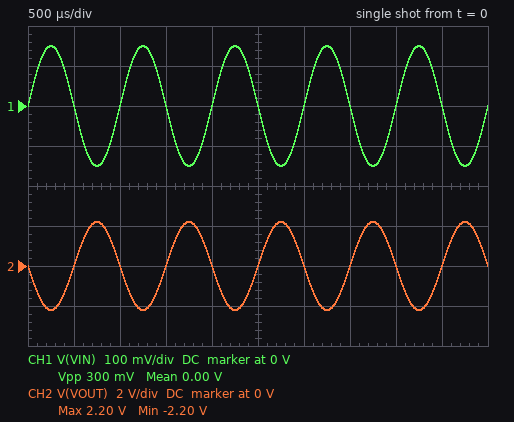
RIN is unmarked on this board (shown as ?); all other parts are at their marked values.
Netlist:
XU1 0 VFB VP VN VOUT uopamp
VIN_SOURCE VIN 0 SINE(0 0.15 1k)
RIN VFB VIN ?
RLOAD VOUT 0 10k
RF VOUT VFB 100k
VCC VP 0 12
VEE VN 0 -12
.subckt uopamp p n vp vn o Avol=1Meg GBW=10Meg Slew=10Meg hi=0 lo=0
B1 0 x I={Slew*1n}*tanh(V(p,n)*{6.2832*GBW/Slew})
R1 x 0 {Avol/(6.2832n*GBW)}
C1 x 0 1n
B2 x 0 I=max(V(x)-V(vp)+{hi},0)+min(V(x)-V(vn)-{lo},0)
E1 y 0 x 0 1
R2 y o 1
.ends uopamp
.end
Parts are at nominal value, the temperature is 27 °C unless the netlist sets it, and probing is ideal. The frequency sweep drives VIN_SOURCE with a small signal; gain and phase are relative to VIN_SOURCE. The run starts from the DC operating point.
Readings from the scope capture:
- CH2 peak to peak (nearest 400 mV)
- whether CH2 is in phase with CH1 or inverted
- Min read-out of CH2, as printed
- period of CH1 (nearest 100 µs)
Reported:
4.4 V
inverted
-2.20 V
1.0 ms
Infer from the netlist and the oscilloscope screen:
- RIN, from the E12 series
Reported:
6.8 kΩ
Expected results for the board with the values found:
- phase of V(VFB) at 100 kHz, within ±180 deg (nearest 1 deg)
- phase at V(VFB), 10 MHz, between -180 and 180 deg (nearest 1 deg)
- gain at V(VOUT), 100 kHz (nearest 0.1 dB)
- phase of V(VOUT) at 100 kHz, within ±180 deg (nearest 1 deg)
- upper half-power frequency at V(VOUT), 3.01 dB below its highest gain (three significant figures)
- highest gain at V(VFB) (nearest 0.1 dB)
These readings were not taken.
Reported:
81 deg
4 deg
23.2 dB
171 deg
637 kHz
-0.6 dB
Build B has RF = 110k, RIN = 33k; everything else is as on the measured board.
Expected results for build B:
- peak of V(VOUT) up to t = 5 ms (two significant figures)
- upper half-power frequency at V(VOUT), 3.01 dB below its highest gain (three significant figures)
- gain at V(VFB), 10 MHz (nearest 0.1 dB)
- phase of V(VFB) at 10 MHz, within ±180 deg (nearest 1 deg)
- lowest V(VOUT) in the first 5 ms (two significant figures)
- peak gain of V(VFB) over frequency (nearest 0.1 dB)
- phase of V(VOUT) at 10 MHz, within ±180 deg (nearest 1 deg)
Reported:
500 mV
2.31 MHz
-2.5 dB
13 deg
-500 mV
-2.3 dB
103 deg
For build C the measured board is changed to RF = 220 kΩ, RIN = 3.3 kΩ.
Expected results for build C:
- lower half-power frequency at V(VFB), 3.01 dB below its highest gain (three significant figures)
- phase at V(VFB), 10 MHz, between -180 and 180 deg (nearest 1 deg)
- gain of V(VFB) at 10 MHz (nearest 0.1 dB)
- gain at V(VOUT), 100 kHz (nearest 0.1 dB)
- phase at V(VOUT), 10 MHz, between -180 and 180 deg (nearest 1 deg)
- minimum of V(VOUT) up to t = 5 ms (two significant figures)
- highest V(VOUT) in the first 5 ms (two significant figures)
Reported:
148 kHz
1 deg
-0.1 dB
34.8 dB
91 deg
-10 V
10 V
